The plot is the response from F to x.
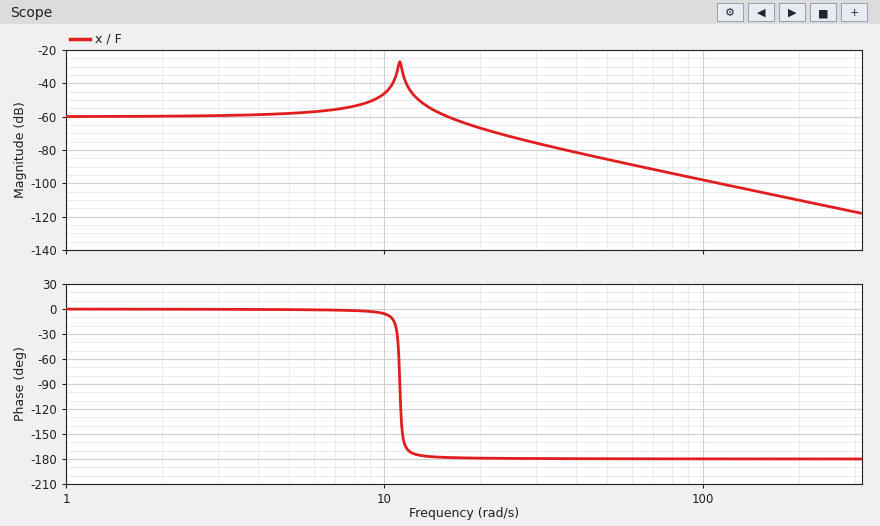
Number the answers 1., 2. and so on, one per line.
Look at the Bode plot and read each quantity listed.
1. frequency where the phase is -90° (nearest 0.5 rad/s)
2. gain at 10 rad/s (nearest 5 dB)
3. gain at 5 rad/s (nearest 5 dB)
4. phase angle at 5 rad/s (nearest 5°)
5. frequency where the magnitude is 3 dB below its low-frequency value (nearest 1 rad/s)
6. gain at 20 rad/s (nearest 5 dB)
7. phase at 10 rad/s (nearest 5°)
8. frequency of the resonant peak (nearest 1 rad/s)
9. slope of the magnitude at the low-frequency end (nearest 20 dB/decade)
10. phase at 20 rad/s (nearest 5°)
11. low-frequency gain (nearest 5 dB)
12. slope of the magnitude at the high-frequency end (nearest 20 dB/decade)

1. 11.0 rad/s
2. -45 dB
3. -60 dB
4. 0°
5. 17 rad/s
6. -65 dB
7. -5°
8. 11 rad/s
9. 0 dB/decade
10. -180°
11. -60 dB
12. -40 dB/decade
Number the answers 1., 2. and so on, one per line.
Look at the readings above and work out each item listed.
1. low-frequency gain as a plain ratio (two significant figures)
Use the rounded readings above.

1. 0.0010
